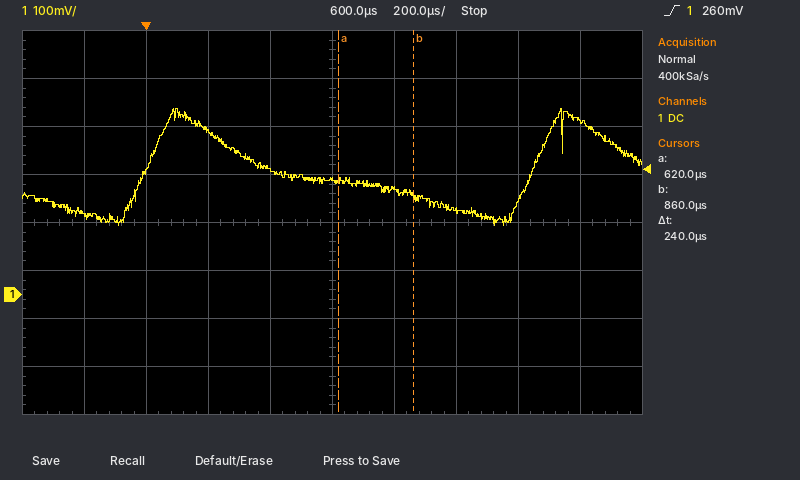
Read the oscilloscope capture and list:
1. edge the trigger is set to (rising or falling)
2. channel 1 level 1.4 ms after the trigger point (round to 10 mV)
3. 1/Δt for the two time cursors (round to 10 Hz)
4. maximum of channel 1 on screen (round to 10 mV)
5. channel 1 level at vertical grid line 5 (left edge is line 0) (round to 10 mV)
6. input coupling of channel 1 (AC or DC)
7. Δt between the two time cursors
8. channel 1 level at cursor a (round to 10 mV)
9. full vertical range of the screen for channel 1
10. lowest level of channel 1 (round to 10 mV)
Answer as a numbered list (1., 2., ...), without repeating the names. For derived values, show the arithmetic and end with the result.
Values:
1. rising
2. 360 mV
3. 1 / 240 µs ≈ 4.17 kHz
4. 390 mV
5. 240 mV
6. DC
7. 240 µs
8. 240 mV
9. 800 mV
10. 140 mV
